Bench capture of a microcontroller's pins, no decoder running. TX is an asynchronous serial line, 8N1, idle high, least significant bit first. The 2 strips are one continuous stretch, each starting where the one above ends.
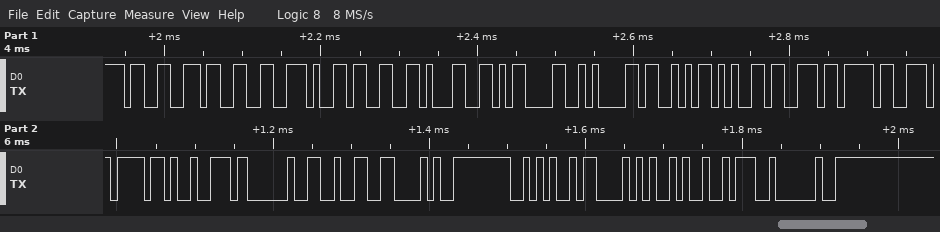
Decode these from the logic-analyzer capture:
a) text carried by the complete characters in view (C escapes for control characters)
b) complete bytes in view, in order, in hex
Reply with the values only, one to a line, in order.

"33.31\r\nSensor 2(*C): "
33 33 2E 33 31 0D 0A 53 65 6E 73 6F 72 20 32 28 2A 43 29 3A 20
